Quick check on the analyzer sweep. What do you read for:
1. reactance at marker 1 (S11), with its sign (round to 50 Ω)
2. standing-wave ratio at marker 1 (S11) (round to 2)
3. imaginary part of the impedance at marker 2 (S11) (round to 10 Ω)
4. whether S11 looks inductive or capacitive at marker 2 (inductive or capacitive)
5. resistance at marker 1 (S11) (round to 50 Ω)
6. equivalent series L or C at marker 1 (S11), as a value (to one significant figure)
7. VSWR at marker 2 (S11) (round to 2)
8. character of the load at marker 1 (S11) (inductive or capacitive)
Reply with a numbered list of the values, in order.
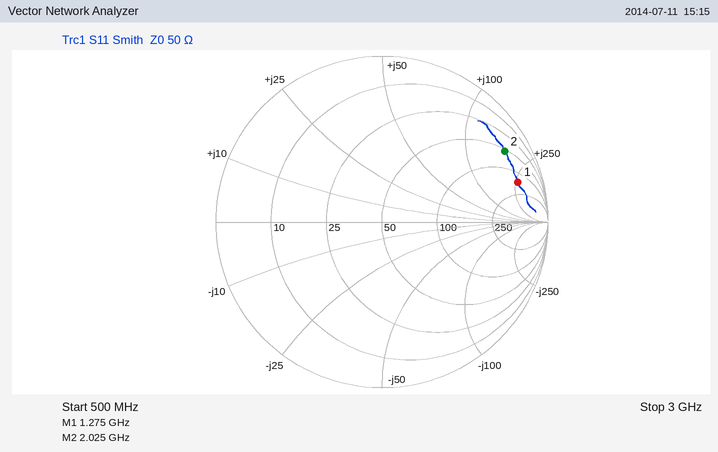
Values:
1. +250 Ω
2. 12
3. +170 Ω
4. inductive
5. 150 Ω
6. 30 nH
7. 12
8. inductive
